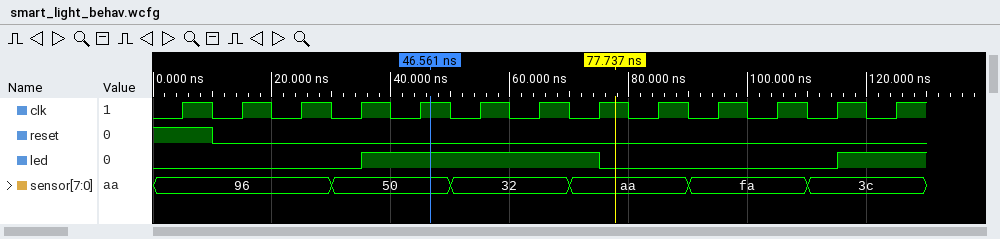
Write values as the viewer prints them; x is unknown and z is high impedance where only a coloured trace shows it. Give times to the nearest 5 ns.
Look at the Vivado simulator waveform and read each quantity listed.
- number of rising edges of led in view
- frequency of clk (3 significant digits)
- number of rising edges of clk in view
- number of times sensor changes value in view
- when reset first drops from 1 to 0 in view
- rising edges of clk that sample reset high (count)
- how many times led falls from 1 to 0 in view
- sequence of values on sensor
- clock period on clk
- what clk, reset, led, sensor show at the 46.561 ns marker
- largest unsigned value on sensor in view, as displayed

2
100 MHz
13
5
10 ns
1
1
96, 50, 32, aa, fa, 3c
10 ns
clk=1, reset=0, led=1, sensor=50
fa
